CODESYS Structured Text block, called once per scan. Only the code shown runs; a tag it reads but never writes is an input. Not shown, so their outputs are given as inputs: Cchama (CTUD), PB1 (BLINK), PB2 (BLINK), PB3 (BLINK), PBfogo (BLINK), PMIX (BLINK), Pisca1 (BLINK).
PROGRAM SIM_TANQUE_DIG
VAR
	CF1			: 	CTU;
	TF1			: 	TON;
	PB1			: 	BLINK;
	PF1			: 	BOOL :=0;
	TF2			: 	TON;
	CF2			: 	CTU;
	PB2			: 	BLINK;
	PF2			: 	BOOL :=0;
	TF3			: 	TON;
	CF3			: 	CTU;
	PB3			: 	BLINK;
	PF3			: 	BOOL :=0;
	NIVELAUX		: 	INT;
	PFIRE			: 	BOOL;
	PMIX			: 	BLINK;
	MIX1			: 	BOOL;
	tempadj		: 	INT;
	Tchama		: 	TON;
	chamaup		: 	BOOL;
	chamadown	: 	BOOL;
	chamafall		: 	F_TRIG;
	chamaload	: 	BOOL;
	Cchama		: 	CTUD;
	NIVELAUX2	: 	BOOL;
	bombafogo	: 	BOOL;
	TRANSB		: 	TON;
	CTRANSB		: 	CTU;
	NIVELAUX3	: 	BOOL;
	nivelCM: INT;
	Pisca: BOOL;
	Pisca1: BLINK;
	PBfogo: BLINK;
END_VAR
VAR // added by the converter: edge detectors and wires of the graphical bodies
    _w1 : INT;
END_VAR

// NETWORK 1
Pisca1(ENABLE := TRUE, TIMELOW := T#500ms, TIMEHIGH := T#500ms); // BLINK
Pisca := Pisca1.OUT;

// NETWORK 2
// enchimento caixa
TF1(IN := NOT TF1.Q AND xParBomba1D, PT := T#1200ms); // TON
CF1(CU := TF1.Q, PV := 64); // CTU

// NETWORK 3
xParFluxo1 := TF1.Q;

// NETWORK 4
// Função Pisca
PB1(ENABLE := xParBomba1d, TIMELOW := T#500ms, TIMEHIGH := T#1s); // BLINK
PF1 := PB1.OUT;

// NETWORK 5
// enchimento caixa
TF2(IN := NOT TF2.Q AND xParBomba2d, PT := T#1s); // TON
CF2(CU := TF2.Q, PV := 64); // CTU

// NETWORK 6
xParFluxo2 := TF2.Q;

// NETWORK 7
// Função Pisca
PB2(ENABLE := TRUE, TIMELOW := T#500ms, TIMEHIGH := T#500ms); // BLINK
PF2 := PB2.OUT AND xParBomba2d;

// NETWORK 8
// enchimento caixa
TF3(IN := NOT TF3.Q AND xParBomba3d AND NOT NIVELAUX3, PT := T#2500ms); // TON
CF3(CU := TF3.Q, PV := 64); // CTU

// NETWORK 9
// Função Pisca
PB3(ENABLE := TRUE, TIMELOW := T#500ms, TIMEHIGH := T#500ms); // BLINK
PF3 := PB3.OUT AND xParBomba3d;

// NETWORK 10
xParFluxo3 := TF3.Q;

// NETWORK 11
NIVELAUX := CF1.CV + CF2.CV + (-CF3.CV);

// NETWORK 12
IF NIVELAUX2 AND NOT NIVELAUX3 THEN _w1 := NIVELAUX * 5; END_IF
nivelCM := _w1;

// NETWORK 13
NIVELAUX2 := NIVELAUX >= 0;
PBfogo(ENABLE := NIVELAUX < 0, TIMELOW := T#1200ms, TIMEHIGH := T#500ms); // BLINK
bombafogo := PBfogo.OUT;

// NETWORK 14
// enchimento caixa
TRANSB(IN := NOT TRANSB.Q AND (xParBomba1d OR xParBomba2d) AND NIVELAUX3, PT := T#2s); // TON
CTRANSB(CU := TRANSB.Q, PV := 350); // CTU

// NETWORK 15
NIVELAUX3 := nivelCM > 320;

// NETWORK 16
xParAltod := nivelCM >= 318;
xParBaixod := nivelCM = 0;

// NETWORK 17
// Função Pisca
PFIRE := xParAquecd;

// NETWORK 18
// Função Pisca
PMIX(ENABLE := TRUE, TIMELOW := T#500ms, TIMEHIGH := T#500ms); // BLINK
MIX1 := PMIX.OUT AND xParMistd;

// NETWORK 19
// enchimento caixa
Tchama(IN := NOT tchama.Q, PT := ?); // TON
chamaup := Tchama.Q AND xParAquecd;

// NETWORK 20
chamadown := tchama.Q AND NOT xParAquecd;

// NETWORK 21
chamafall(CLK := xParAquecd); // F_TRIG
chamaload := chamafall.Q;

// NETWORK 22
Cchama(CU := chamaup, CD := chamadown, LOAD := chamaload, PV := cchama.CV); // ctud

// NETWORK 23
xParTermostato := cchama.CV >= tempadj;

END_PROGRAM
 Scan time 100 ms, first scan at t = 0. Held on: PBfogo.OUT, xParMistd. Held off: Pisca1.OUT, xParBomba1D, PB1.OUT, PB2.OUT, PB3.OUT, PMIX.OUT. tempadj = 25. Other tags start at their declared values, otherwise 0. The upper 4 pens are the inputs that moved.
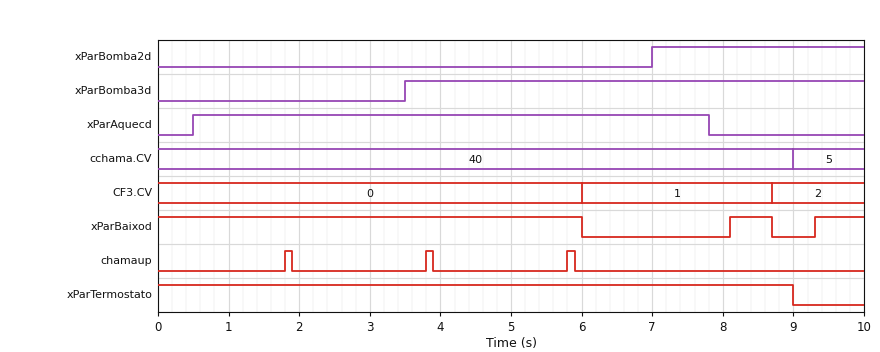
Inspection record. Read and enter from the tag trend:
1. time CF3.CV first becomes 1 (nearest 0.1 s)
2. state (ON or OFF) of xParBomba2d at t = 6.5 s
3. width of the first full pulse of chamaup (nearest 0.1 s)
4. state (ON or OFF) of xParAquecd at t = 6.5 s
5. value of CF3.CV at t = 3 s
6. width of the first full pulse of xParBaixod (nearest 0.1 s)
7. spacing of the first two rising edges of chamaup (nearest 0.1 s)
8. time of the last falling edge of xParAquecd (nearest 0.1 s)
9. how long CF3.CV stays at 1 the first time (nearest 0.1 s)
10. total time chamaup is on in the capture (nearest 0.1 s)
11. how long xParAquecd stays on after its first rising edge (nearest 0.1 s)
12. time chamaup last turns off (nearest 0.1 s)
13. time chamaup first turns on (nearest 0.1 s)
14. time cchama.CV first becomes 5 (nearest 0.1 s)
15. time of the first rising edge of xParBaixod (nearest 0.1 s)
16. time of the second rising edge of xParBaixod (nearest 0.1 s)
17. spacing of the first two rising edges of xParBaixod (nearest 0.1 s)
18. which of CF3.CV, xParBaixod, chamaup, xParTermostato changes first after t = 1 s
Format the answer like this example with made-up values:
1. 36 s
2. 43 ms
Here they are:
1. 6.0 s
2. OFF
3. 0.1 s
4. ON
5. 0
6. 0.6 s
7. 2.0 s
8. 7.8 s
9. 2.7 s
10. 0.3 s
11. 7.3 s
12. 5.9 s
13. 1.8 s
14. 9.0 s
15. 8.1 s
16. 9.3 s
17. 1.2 s
18. chamaup
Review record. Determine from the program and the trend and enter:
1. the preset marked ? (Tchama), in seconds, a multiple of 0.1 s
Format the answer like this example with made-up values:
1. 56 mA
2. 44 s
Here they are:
1. 1.8 s
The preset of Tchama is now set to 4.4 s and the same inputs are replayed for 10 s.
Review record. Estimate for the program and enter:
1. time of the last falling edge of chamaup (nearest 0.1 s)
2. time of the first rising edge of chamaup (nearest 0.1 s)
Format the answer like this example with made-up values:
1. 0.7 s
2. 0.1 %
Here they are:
1. 4.5 s
2. 4.4 s
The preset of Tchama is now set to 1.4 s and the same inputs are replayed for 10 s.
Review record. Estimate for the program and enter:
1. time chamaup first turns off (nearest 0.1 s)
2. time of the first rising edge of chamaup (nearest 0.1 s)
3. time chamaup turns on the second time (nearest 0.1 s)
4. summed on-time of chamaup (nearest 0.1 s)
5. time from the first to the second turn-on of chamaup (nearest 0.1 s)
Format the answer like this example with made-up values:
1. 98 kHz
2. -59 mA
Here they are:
1. 1.5 s
2. 1.4 s
3. 3.0 s
4. 0.4 s
5. 1.6 s
